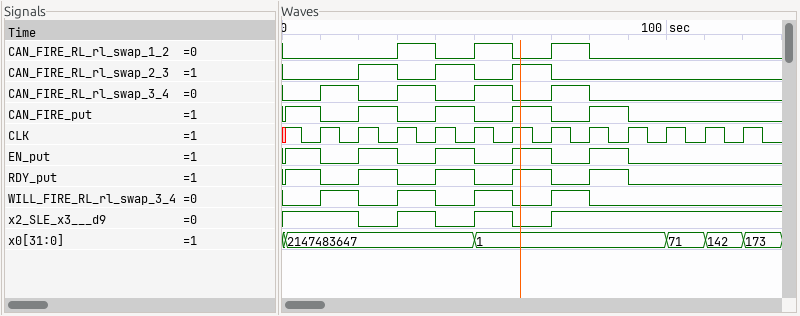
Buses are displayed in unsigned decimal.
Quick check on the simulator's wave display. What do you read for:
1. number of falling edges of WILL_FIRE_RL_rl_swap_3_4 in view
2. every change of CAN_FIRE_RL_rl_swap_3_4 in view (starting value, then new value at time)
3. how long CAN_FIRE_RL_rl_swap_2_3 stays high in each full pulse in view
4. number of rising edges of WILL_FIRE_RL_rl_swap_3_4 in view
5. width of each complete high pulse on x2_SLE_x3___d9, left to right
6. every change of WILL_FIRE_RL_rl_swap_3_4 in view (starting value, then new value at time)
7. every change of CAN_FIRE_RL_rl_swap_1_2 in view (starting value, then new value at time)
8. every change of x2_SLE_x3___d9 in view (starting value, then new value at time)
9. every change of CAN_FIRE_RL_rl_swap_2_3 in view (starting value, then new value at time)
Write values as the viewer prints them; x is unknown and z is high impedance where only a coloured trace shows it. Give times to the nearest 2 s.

4
0, 1 at 10 s, 0 at 20 s, 1 at 30 s, 0 at 40 s, 1 at 50 s, 0 at 60 s, 1 at 70 s, 0 at 80 s
10 s, 10 s, 10 s
4
10 s, 10 s
0, 1 at 10 s, 0 at 20 s, 1 at 30 s, 0 at 40 s, 1 at 50 s, 0 at 60 s, 1 at 70 s, 0 at 80 s
0, 1 at 30 s, 0 at 40 s, 1 at 50 s, 0 at 60 s, 1 at 70 s, 0 at 80 s
1, 0 at 20 s, 1 at 30 s, 0 at 40 s, 1 at 50 s, 0 at 60 s, 1 at 70 s
0, 1 at 20 s, 0 at 30 s, 1 at 40 s, 0 at 50 s, 1 at 60 s, 0 at 70 s
